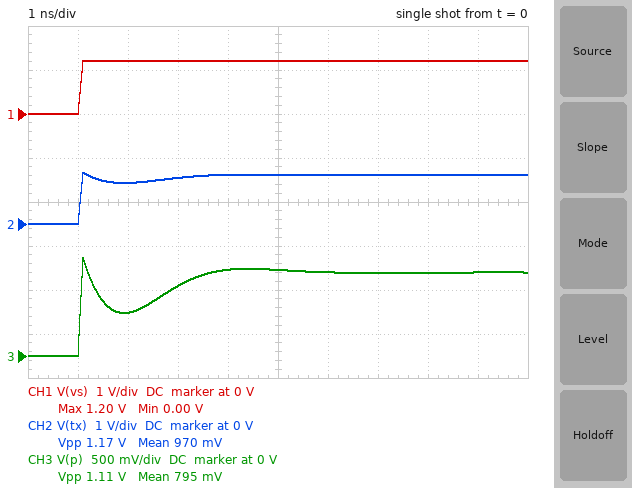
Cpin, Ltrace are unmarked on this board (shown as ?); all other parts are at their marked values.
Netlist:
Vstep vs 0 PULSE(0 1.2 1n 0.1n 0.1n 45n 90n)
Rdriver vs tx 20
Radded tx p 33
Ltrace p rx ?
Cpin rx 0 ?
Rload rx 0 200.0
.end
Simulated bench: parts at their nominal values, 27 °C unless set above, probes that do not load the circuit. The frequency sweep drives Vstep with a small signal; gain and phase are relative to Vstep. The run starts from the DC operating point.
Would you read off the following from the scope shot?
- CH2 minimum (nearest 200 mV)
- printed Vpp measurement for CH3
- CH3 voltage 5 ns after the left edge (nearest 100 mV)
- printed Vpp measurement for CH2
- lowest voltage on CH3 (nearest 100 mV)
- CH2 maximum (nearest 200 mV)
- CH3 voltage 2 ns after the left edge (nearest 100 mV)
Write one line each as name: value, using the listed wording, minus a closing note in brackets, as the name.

CH2 minimum: 0 V
printed Vpp measurement for CH3: 1.11 V
CH3 voltage 5 ns after the left edge: 1.0 V
printed Vpp measurement for CH2: 1.17 V
lowest voltage on CH3: 0 V
CH2 maximum: 1.2 V
CH3 voltage 2 ns after the left edge: 500 mV
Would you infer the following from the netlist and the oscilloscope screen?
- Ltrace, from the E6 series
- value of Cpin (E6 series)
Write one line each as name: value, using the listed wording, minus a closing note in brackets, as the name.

Ltrace, from the E6 series: 33 nH
value of Cpin: 15 pF
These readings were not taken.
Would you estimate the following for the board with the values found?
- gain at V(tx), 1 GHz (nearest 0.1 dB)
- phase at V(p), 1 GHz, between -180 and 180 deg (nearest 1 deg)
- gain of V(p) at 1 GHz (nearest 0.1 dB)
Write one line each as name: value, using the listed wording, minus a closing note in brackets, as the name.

gain at V(tx), 1 GHz: -0.2 dB
phase at V(p), 1 GHz, between -180 and 180 deg: 15 deg
gain of V(p) at 1 GHz: -0.3 dB
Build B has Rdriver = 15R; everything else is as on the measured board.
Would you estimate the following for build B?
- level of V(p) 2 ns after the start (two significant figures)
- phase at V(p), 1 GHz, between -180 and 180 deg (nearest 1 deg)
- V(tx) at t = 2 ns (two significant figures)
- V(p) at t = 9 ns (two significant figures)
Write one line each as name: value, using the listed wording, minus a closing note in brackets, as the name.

level of V(p) 2 ns after the start: 520 mV
phase at V(p), 1 GHz, between -180 and 180 deg: 14 deg
V(tx) at t = 2 ns: 990 mV
V(p) at t = 9 ns: 970 mV
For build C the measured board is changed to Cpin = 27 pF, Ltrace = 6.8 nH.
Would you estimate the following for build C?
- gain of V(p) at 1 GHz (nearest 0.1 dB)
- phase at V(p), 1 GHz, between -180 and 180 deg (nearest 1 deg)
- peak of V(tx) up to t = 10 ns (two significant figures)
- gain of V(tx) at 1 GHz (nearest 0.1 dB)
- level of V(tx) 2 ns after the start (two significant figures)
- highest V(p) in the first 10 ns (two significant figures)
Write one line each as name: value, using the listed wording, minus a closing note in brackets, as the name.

gain of V(p) at 1 GHz: -4.9 dB
phase at V(p), 1 GHz, between -180 and 180 deg: 55 deg
peak of V(tx) up to t = 10 ns: 1.1 V
gain of V(tx) at 1 GHz: -2.3 dB
level of V(tx) 2 ns after the start: 920 mV
highest V(p) in the first 10 ns: 950 mV
